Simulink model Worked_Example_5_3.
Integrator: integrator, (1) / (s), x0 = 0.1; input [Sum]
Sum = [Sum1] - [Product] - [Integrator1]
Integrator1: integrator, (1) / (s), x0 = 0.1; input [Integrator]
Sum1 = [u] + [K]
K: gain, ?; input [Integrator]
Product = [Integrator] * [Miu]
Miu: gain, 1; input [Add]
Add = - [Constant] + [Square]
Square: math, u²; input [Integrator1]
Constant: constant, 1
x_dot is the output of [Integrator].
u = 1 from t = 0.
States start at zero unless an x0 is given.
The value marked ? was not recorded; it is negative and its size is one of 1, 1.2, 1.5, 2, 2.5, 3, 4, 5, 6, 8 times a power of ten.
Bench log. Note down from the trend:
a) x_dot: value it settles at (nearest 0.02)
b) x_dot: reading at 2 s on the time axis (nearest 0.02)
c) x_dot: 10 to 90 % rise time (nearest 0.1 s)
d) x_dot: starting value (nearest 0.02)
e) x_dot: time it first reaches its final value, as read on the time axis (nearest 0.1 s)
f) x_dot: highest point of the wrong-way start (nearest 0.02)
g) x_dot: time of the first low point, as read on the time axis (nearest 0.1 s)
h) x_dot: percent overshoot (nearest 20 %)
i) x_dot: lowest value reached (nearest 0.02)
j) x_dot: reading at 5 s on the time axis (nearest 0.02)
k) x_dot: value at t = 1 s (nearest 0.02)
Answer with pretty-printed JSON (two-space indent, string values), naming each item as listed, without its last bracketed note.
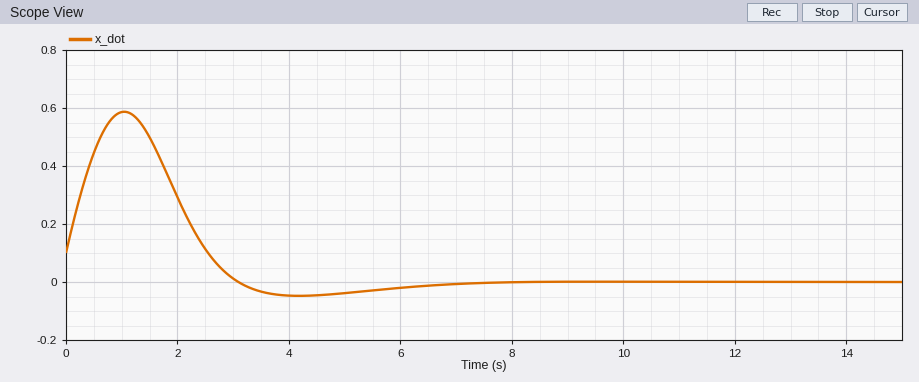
{
  "x_dot: value it settles at": "0.00",
  "x_dot: reading at 2 s on the time axis": "0.30",
  "x_dot: 10 to 90 % rise time": "0.4 s",
  "x_dot: starting value": "0.10",
  "x_dot: time it first reaches its final value, as read on the time axis": "3.1 s",
  "x_dot: highest point of the wrong-way start": "0.58",
  "x_dot: time of the first low point, as read on the time axis": "4.2 s",
  "x_dot: percent overshoot": "40 %",
  "x_dot: lowest value reached": "-0.04",
  "x_dot: reading at 5 s on the time axis": "-0.04",
  "x_dot: value at t = 1 s": "0.58"
}
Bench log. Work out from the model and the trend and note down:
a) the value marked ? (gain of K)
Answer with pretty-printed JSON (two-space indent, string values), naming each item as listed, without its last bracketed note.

{
  "the value marked ?": "-1.5"
}
